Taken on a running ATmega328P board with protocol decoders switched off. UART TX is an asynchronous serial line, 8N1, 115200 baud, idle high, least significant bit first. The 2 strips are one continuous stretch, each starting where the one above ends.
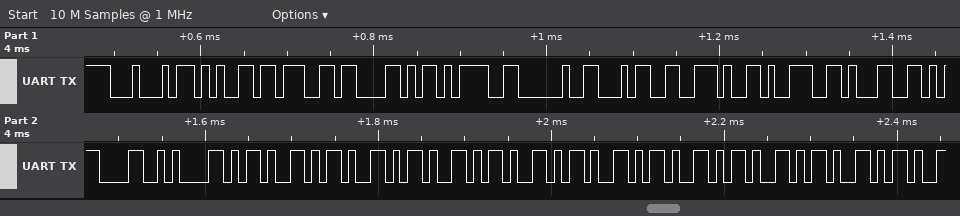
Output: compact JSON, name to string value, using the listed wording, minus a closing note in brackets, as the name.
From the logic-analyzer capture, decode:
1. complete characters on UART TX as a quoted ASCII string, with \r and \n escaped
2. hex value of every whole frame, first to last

{"complete characters on UART TX as a quoted ASCII string, with \\r and \\n escaped": "\"DegX= 4.91\\r\\n---------\"", "hex value of every whole frame, first to last": "44 65 67 58 3D 20 34 2E 39 31 0D 0A 2D 2D 2D 2D 2D 2D 2D 2D 2D"}
